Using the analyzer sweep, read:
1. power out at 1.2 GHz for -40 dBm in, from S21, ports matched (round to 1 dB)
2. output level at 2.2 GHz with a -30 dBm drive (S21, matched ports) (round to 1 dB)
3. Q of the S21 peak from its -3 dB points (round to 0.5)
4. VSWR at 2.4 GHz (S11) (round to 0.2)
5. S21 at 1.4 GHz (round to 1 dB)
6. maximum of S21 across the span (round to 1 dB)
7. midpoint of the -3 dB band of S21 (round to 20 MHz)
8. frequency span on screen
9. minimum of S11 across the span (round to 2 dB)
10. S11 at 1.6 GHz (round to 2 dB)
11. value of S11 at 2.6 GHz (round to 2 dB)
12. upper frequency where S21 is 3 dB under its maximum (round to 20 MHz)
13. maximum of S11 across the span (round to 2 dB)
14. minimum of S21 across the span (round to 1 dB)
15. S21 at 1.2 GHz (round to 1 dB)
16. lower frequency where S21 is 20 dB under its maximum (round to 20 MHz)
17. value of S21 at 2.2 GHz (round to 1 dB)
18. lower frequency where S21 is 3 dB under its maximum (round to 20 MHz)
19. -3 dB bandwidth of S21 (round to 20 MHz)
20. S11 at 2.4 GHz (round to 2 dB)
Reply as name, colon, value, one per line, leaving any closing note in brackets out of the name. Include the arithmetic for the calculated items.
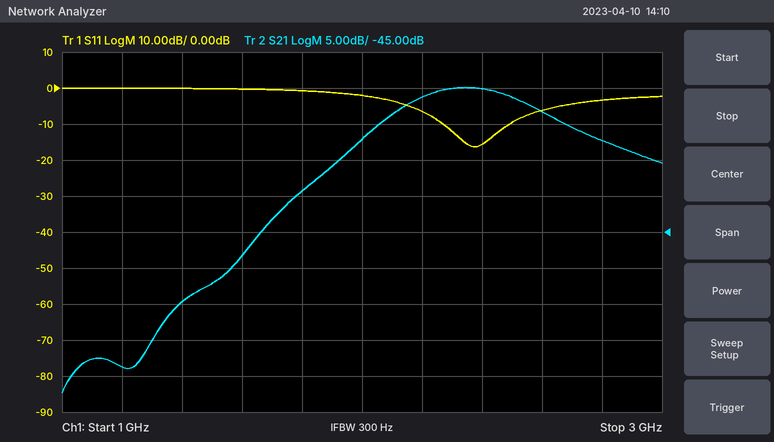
power out at 1.2 GHz for -40 dBm in, from S21, ports matched: -40 dBm + (-64 dB) = -104 dBm
output level at 2.2 GHz with a -30 dBm drive (S21, matched ports): -30 dBm + (-26 dB) = -56 dBm
Q of the S21 peak from its -3 dB points: 2.35 GHz / 460 MHz ≈ 5.11, so 5.0 to the nearest 0.5
VSWR at 2.4 GHz (S11): |Γ| = 10^(-16/20) = 0.1585; VSWR = (1 + 0.1585)/(1 − 0.1585) ≈ 1.4
S21 at 1.4 GHz: -55 dB
maximum of S21 across the span: -25 dB
midpoint of the -3 dB band of S21: 2.36 GHz
frequency span on screen: 2 GHz
minimum of S11 across the span: -16 dB
S11 at 1.6 GHz: 0 dB
value of S11 at 2.6 GHz: -6 dB
upper frequency where S21 is 3 dB under its maximum: 2.58 GHz
maximum of S11 across the span: 0 dB
minimum of S21 across the span: -67 dB
S21 at 1.2 GHz: -64 dB
lower frequency where S21 is 20 dB under its maximum: 1.66 GHz
value of S21 at 2.2 GHz: -26 dB
lower frequency where S21 is 3 dB under its maximum: 2.12 GHz
-3 dB bandwidth of S21: 2.58 GHz − 2.12 GHz = 460 MHz
S11 at 2.4 GHz: -16 dB
